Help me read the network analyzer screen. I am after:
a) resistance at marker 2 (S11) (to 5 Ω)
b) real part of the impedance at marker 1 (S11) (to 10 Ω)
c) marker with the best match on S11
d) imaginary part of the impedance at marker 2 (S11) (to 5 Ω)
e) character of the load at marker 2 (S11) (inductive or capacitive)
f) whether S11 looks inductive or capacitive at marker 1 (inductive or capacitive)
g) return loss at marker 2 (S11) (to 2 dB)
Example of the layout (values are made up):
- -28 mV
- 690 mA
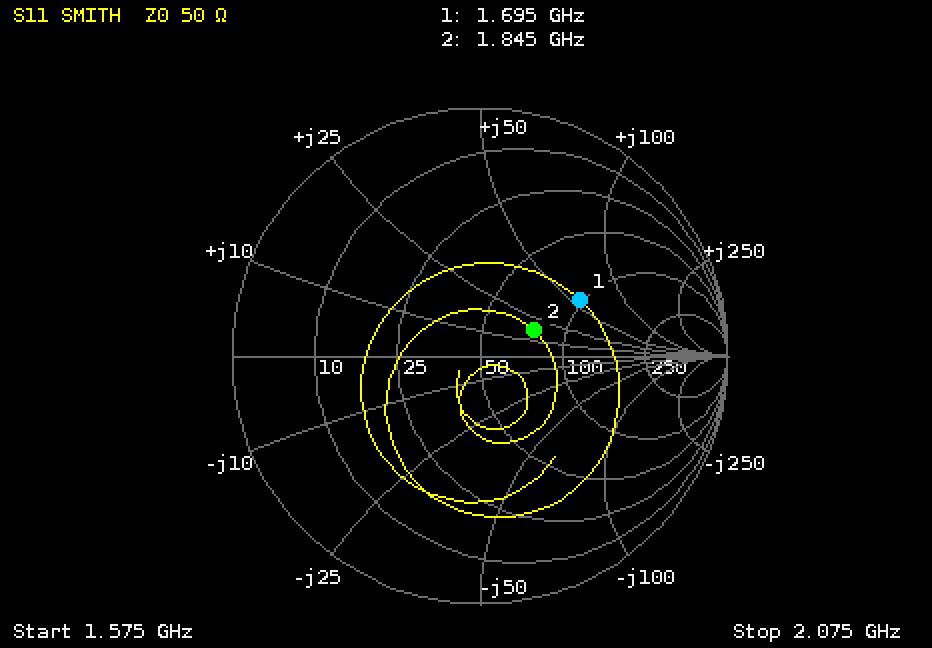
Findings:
- 75 Ω
- 100 Ω
- marker 2
- +15 Ω
- inductive
- inductive
- 12 dB
